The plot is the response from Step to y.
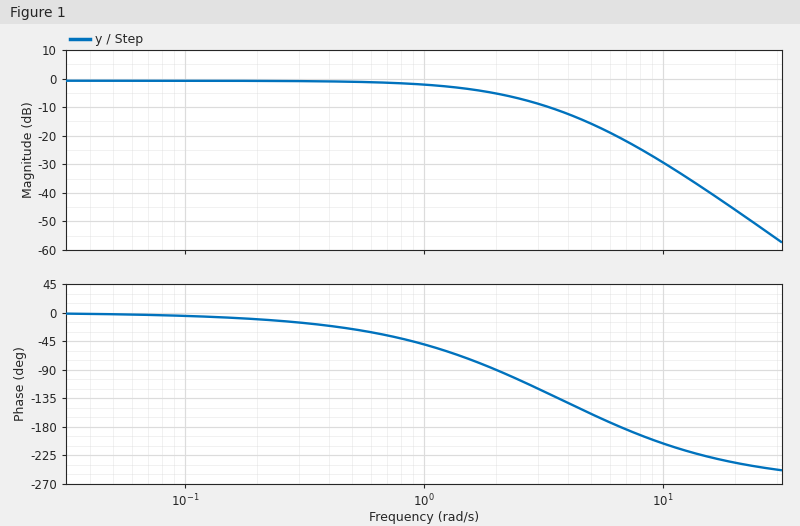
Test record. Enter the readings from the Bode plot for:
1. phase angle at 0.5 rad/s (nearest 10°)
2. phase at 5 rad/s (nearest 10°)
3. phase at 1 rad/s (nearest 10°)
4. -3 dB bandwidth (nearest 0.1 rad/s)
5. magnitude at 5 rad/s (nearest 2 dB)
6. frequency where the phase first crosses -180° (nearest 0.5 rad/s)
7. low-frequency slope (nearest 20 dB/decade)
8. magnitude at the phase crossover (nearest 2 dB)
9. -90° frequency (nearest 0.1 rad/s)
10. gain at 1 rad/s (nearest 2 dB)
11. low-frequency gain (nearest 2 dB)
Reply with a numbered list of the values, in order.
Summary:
1. -30°
2. -160°
3. -50°
4. 1.6 rad/s
5. -16 dB
6. 6.5 rad/s
7. 0 dB/decade
8. -20 dB
9. 2.0 rad/s
10. -2 dB
11. 0 dB
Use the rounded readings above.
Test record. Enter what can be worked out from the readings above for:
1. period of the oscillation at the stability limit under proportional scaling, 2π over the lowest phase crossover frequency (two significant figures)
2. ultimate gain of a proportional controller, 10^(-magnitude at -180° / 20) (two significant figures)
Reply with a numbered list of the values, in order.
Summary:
1. 0.97 s
2. 10
